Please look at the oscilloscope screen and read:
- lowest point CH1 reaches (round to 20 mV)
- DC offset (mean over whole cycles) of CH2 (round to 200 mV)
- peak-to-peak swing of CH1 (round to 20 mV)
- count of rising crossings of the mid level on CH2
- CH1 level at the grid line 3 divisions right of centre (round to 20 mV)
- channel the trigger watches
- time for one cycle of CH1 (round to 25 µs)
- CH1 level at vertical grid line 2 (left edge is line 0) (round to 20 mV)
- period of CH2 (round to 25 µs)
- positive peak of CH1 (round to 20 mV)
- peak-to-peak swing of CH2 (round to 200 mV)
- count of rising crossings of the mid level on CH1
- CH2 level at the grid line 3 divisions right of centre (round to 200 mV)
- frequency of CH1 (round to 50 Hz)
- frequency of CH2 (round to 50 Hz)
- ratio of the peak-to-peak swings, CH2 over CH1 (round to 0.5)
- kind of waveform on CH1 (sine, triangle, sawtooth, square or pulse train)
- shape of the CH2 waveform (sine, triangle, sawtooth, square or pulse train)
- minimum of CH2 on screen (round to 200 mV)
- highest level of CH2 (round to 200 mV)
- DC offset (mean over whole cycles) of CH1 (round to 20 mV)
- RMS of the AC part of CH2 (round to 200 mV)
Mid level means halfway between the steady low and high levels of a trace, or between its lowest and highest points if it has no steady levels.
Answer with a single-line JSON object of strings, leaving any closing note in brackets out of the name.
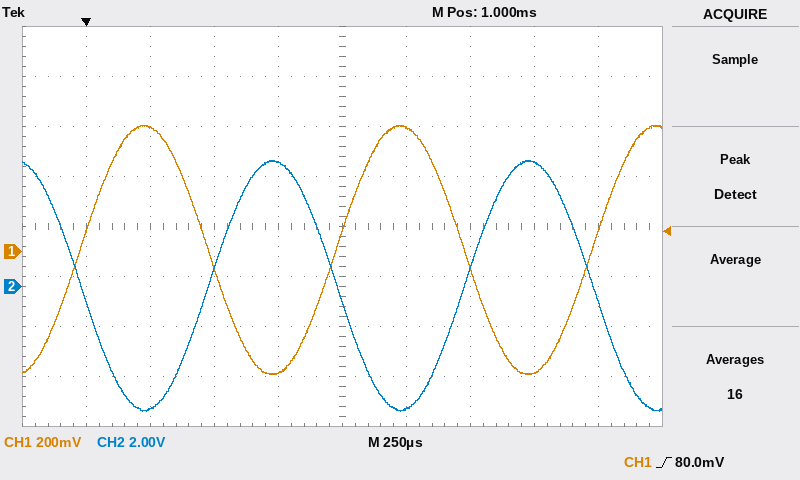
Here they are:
{"lowest point CH1 reaches": "-500 mV", "DC offset (mean over whole cycles) of CH2": "0.0 V", "peak-to-peak swing of CH1": "1.00 V", "count of rising crossings of the mid level on CH2": "2", "CH1 level at the grid line 3 divisions right of centre": "-480 mV", "channel the trigger watches": "CH1", "time for one cycle of CH1": "1.000 ms", "CH1 level at vertical grid line 2 (left edge is line 0)": "500 mV", "period of CH2": "1.000 ms", "positive peak of CH1": "500 mV", "peak-to-peak swing of CH2": "10.0 V", "count of rising crossings of the mid level on CH1": "3", "CH2 level at the grid line 3 divisions right of centre": "5.0 V", "frequency of CH1": "1.00 kHz", "frequency of CH2": "1.00 kHz", "ratio of the peak-to-peak swings, CH2 over CH1": "10.0", "kind of waveform on CH1": "sine", "shape of the CH2 waveform": "sine", "minimum of CH2 on screen": "-5.0 V", "highest level of CH2": "5.0 V", "DC offset (mean over whole cycles) of CH1": "0 mV", "RMS of the AC part of CH2": "3.6 V"}
